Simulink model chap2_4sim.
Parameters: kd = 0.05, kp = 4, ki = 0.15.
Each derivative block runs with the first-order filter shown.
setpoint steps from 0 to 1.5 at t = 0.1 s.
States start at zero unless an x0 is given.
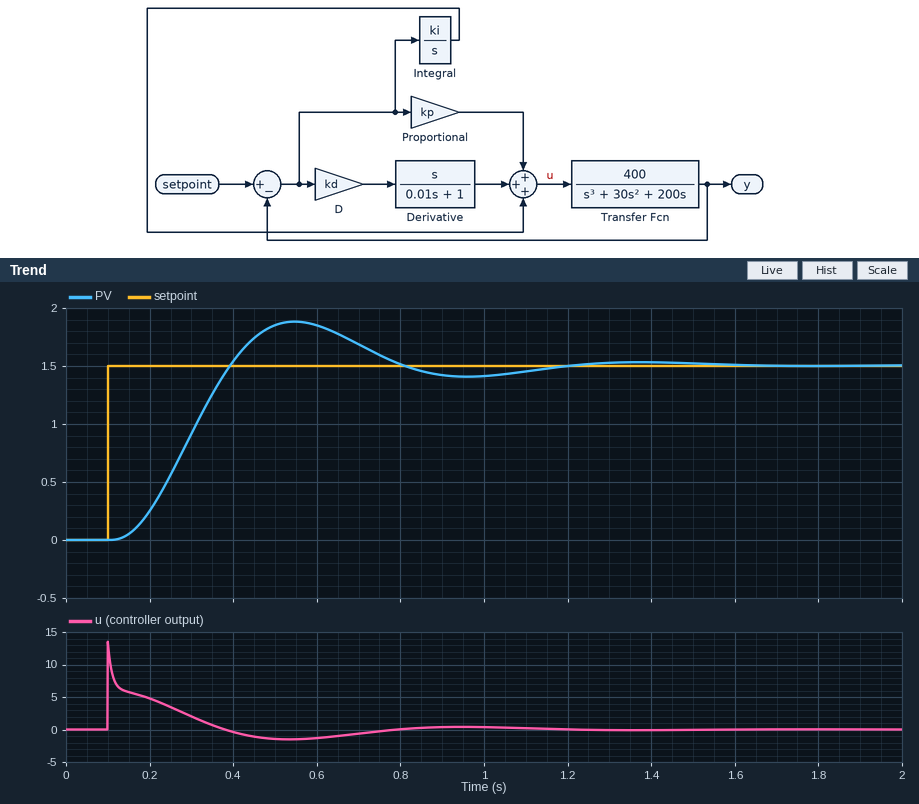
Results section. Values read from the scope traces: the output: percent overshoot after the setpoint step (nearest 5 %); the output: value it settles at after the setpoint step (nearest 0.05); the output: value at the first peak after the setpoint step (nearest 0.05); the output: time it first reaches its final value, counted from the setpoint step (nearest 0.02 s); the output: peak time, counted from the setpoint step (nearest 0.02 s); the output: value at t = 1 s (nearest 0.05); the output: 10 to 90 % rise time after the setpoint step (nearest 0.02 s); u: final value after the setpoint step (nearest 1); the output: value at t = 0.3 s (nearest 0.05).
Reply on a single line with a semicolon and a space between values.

25 %; 1.50; 1.90; 0.30 s; 0.44 s; 1.40; 0.18 s; 0; 0.90
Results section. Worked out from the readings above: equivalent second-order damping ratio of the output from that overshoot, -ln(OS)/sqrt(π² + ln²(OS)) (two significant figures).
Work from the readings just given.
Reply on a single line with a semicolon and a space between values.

0.40
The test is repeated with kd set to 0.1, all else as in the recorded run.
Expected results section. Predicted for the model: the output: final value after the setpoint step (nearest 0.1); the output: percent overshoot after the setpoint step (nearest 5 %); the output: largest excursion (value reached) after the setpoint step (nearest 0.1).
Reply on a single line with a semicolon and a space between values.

1.5; 20 %; 1.8
